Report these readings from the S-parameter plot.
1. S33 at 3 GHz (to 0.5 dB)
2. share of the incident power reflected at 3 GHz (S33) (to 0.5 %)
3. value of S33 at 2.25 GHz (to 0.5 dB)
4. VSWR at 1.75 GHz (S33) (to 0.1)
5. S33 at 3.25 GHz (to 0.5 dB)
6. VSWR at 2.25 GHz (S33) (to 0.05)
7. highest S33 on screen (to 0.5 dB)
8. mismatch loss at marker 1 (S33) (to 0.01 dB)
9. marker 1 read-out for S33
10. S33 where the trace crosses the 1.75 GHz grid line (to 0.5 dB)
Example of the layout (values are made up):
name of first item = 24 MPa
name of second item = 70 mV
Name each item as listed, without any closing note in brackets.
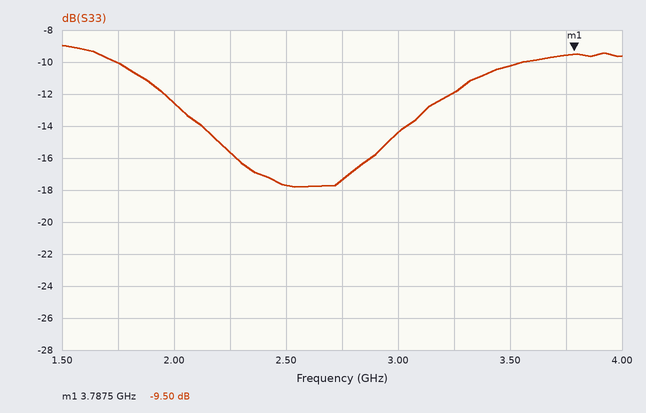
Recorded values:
S33 at 3 GHz = -14.5 dB
share of the incident power reflected at 3 GHz (S33) = 3.5 %
value of S33 at 2.25 GHz = -15.5 dB
VSWR at 1.75 GHz (S33) = 1.9
S33 at 3.25 GHz = -12.0 dB
VSWR at 2.25 GHz (S33) = 1.40
highest S33 on screen = -9.0 dB
mismatch loss at marker 1 (S33) = 0.52 dB
marker 1 read-out for S33 = -9.50 dB
S33 where the trace crosses the 1.75 GHz grid line = -10.0 dB
